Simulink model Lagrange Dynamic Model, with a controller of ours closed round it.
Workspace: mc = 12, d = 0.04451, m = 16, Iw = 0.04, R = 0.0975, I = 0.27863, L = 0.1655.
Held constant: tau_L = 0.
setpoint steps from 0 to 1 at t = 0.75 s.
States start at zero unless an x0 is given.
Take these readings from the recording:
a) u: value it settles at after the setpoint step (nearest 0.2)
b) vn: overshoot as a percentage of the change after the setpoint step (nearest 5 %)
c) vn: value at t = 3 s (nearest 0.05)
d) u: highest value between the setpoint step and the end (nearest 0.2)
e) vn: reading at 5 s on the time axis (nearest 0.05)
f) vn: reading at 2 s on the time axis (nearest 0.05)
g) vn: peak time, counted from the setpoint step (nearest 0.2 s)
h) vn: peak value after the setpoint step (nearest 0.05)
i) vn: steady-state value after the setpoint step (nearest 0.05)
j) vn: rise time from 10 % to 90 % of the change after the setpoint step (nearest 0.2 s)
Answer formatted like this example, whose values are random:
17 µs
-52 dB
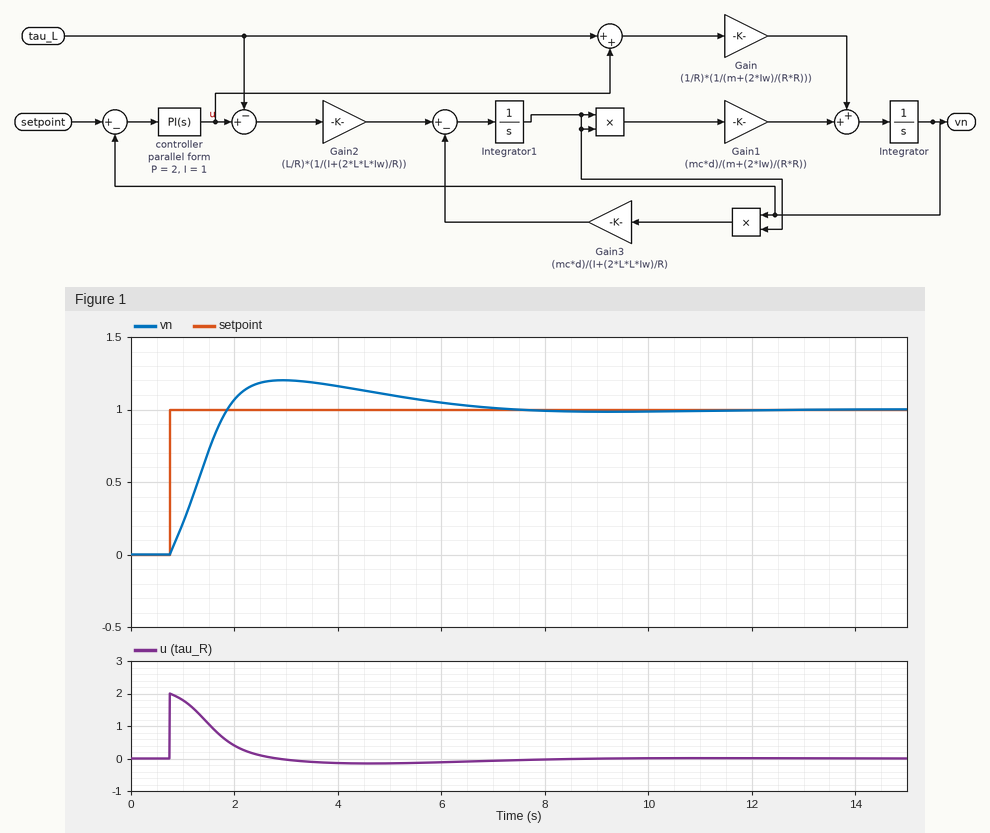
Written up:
0.0
20 %
1.20
2.0
1.10
1.05
2.2 s
1.20
1.00
0.8 s
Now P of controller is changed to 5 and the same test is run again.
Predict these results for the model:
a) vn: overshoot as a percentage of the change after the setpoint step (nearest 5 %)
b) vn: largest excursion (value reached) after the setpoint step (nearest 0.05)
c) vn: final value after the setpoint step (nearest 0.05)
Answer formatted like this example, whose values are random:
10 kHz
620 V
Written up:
10 %
1.10
1.00
